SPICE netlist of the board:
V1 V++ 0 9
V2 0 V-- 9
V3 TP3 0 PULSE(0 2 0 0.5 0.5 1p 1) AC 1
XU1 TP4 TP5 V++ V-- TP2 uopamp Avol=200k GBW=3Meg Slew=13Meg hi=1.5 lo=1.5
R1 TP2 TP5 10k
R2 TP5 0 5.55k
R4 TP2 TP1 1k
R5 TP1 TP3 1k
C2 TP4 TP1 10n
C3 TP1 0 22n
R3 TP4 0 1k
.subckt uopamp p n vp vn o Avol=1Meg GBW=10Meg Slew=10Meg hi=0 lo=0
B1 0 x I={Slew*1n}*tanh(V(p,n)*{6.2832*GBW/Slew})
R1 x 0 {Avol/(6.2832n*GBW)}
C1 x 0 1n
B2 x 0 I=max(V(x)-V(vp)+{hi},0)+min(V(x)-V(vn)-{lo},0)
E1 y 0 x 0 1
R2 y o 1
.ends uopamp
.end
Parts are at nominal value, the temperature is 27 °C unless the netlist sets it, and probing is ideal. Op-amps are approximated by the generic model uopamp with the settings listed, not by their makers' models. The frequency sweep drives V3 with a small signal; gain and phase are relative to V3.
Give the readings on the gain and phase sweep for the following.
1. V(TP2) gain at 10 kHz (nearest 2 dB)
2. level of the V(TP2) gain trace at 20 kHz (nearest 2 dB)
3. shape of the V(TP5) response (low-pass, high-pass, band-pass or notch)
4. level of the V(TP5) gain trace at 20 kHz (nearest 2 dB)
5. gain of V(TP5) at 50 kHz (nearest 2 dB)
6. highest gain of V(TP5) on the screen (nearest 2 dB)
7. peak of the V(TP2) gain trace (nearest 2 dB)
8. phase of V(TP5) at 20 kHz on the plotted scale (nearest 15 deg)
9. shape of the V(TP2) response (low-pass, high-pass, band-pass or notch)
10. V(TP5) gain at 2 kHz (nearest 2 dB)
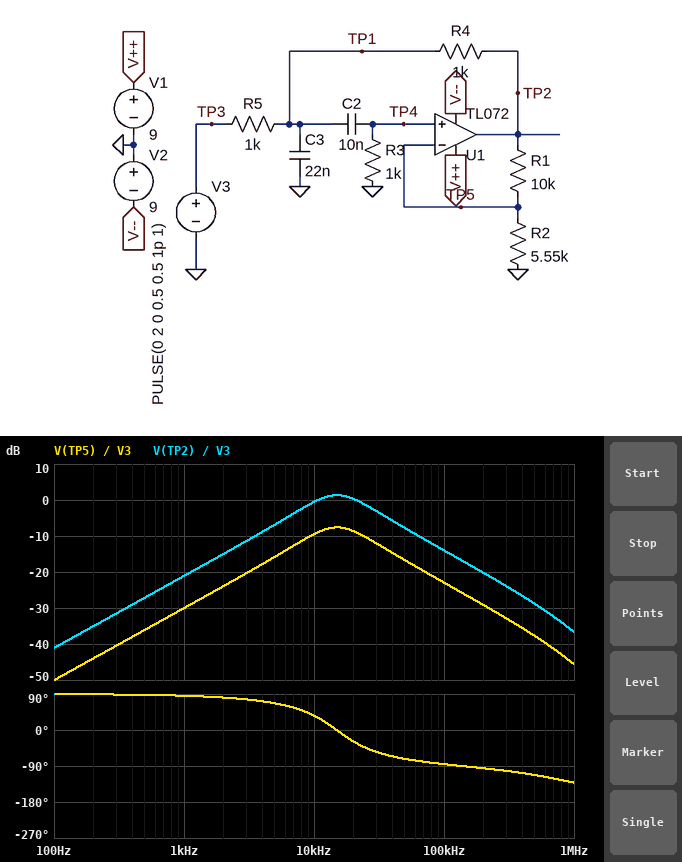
0 dB
0 dB
band-pass
-8 dB
-16 dB
-8 dB
2 dB
-30 deg
band-pass
-24 dB
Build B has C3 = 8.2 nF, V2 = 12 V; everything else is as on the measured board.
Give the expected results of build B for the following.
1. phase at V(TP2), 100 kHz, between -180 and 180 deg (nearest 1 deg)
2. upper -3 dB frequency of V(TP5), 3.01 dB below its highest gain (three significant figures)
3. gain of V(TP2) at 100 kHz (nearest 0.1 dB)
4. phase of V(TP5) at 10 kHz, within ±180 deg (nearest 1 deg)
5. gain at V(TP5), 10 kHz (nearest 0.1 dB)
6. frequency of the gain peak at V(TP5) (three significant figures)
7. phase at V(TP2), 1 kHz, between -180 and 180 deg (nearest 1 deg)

-84 deg
35.4 kHz
-5.4 dB
68 deg
-9.0 dB
24.2 kHz
88 deg
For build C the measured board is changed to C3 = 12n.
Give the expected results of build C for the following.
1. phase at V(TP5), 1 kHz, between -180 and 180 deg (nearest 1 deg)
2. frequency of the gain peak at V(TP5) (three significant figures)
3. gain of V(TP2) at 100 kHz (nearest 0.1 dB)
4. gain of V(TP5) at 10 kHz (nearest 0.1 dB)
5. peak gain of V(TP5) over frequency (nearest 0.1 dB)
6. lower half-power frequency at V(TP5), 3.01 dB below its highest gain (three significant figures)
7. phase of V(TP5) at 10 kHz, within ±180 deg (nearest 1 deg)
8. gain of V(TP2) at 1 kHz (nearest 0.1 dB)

87 deg
20.2 kHz
-8.7 dB
-8.9 dB
-2.9 dB
13.1 kHz
59 deg
-21.1 dB
